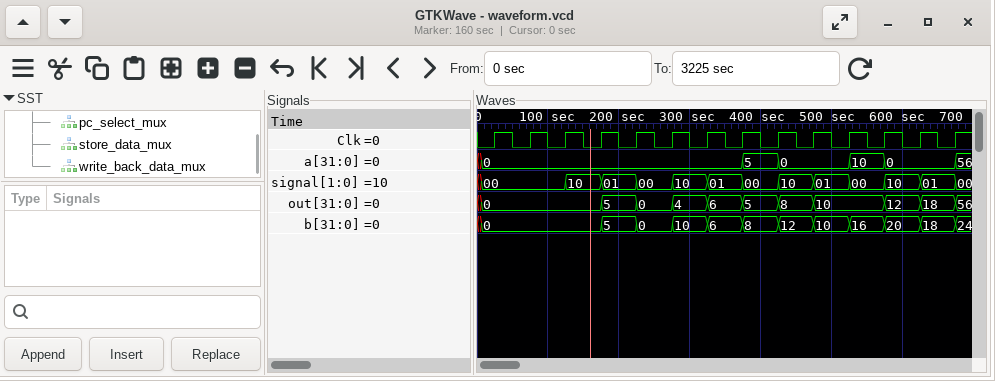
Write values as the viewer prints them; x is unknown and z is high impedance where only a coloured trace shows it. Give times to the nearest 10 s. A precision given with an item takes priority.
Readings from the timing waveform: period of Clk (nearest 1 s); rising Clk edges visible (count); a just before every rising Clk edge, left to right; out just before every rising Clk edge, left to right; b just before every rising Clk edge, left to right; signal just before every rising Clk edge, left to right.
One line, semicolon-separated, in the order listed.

50 s; 14; 0, 0, 0, 0, 0, 0, 0, 0, 5, 0, 0, 10, 0, 0; 0, 0, 0, 0, 5, 0, 4, 6, 5, 8, 10, 10, 12, 18; 0, 0, 0, 0, 5, 0, 10, 6, 8, 12, 10, 16, 20, 18; 00, 00, 00, 10, 01, 00, 10, 01, 00, 10, 01, 00, 10, 01
